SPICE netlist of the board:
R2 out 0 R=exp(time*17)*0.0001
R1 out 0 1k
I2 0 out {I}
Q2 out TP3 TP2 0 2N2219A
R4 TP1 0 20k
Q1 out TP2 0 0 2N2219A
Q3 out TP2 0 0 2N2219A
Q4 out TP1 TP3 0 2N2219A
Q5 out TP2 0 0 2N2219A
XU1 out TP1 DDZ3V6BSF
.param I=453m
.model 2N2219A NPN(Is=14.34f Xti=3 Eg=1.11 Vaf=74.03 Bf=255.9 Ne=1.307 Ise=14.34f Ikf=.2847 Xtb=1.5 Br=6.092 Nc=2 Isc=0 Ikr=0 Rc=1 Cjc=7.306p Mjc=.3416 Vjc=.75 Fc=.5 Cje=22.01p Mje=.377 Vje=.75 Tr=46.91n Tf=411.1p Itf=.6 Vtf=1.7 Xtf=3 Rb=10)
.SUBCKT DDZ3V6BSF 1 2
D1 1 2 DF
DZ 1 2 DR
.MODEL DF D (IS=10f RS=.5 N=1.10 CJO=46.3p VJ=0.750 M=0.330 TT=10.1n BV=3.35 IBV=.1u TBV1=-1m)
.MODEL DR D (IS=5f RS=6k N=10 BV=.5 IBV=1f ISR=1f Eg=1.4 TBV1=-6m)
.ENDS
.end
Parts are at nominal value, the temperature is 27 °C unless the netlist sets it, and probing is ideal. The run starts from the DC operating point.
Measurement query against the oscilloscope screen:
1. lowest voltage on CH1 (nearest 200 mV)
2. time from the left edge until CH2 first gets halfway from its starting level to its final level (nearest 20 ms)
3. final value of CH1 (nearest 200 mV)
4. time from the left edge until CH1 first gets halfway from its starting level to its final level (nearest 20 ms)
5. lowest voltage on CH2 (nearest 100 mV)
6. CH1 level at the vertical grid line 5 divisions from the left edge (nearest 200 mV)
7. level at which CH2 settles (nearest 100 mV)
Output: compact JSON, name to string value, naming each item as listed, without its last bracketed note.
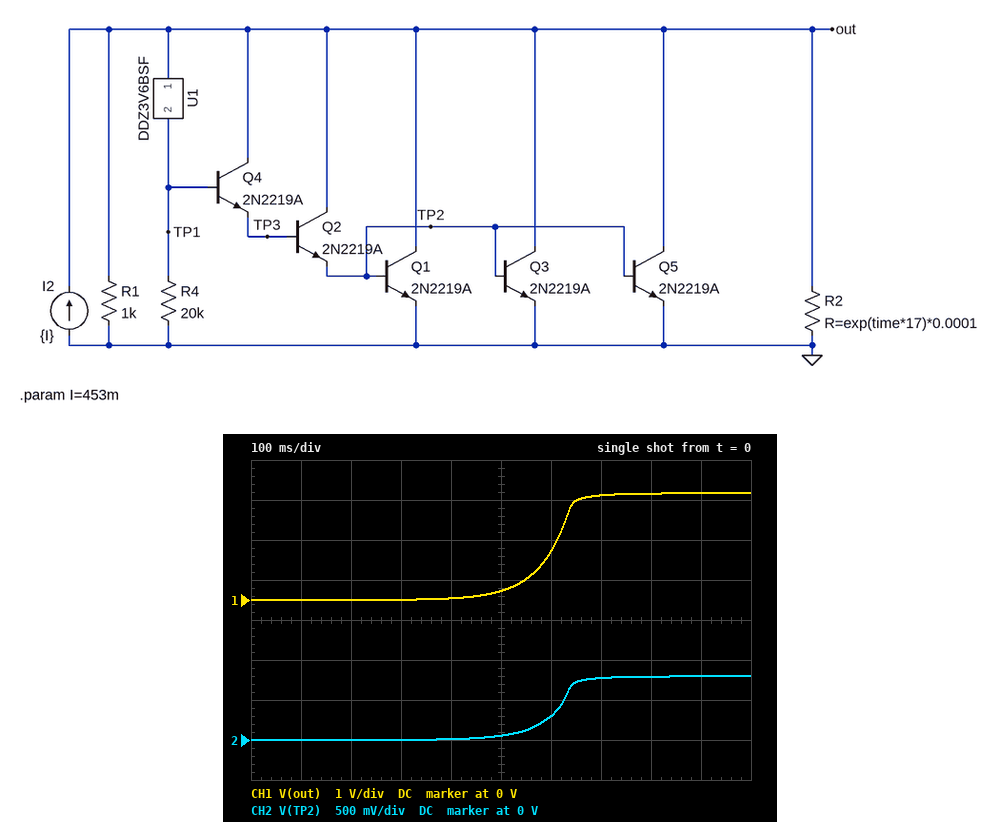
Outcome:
{"lowest voltage on CH1": "0 V", "time from the left edge until CH2 first gets halfway from its starting level to its final level": "620 ms", "final value of CH1": "2.6 V", "time from the left edge until CH1 first gets halfway from its starting level to its final level": "600 ms", "lowest voltage on CH2": "0 V", "CH1 level at the vertical grid line 5 divisions from the left edge": "200 mV", "level at which CH2 settles": "800 mV"}
